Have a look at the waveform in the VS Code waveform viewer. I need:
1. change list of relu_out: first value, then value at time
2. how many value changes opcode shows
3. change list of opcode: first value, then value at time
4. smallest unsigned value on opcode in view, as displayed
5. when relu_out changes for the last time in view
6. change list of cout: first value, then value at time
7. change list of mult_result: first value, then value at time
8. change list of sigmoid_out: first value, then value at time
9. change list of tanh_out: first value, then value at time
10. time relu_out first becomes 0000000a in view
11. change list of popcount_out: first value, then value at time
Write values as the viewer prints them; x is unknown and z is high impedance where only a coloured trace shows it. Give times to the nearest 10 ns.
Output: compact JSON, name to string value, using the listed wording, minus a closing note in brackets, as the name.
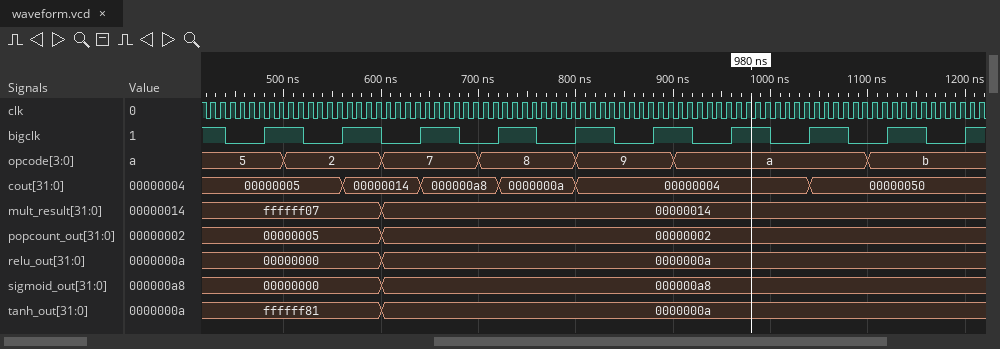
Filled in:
{"change list of relu_out: first value, then value at time": "00000000, 0000000a at 600 ns", "how many value changes opcode shows": "6", "change list of opcode: first value, then value at time": "5, 2 at 500 ns, 7 at 600 ns, 8 at 700 ns, 9 at 800 ns, a at 900 ns, b at 1100 ns", "smallest unsigned value on opcode in view, as displayed": "2", "when relu_out changes for the last time in view": "600 ns", "change list of cout: first value, then value at time": "00000005, 00000014 at 560 ns, 000000a8 at 640 ns, 0000000a at 720 ns, 00000004 at 800 ns, 00000050 at 1040 ns", "change list of mult_result: first value, then value at time": "ffffff07, 00000014 at 600 ns", "change list of sigmoid_out: first value, then value at time": "00000000, 000000a8 at 600 ns", "change list of tanh_out: first value, then value at time": "ffffff81, 0000000a at 600 ns", "time relu_out first becomes 0000000a in view": "600 ns", "change list of popcount_out: first value, then value at time": "00000005, 00000002 at 600 ns"}
